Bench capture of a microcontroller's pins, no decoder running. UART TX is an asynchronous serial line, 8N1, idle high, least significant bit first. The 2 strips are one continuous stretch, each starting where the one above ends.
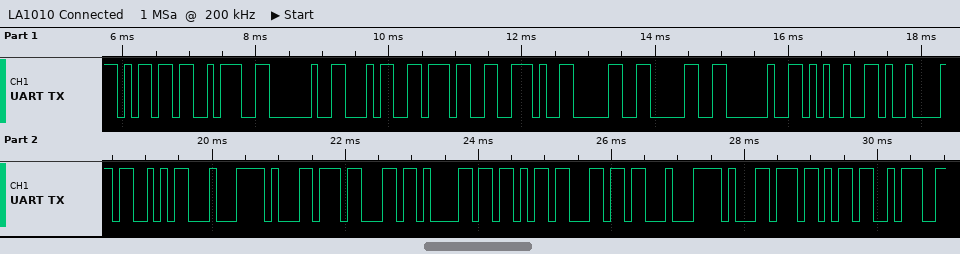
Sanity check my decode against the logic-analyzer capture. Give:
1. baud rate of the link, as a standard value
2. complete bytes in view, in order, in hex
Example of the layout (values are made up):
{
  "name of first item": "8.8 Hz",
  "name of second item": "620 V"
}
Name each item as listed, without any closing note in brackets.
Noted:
{
  "baud rate of the link, as a standard value": "9600 baud",
  "complete bytes in view, in order, in hex": "6D 3A 20 34 37 2E 30 30 20 25 09 53 C4 B1 63 61 6B 6C C4 B1 6B 3A"
}
